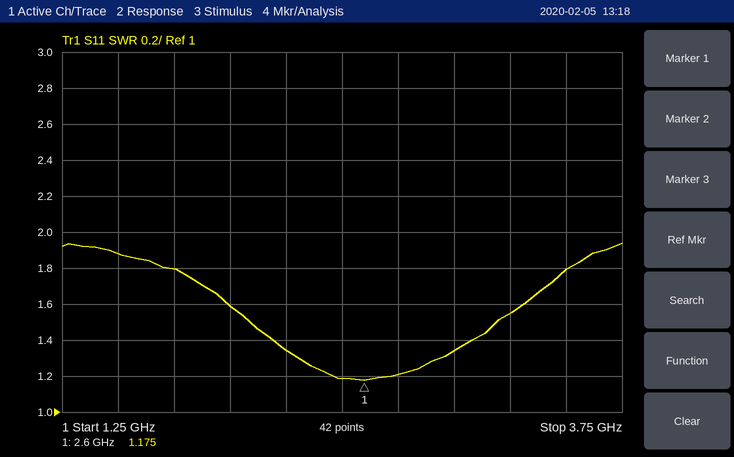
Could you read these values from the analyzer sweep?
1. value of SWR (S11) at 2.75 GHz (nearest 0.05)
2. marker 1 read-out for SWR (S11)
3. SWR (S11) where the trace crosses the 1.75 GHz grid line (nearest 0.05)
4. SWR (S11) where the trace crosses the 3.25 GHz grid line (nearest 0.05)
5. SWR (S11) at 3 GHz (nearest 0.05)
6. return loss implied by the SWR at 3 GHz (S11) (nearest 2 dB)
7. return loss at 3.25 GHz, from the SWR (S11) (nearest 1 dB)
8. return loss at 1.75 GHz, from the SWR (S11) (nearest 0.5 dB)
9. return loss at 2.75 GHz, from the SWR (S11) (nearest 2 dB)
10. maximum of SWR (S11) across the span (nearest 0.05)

1.20
1.175
1.80
1.55
1.35
16 dB
13 dB
11.0 dB
20 dB
1.95
